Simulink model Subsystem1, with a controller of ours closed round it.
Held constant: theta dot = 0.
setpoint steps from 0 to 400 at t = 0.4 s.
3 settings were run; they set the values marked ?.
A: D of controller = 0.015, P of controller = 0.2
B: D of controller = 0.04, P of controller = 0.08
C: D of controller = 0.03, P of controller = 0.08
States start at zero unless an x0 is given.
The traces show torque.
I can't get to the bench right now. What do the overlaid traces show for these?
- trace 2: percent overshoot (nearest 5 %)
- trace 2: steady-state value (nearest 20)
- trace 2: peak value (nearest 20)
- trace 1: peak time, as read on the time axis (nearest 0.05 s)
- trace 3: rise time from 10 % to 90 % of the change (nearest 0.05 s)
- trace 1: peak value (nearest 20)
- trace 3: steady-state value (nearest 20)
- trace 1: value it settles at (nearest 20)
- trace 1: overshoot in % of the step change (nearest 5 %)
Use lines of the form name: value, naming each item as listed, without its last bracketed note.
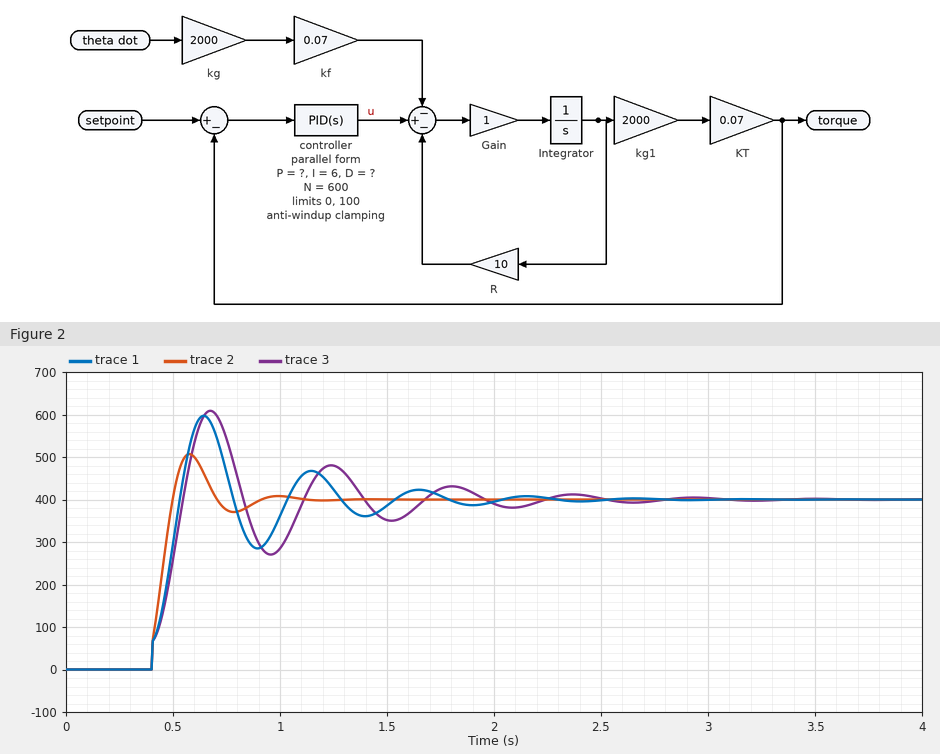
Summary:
trace 2: percent overshoot: 25 %
trace 2: steady-state value: 400
trace 2: peak value: 500
trace 1: peak time, as read on the time axis: 0.65 s
trace 3: rise time from 10 % to 90 % of the change: 0.15 s
trace 1: peak value: 600
trace 3: steady-state value: 400
trace 1: value it settles at: 400
trace 1: overshoot in % of the step change: 50 %
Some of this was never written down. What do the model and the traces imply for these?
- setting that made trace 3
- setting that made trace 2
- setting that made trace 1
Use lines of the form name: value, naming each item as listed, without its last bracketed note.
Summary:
setting that made trace 3: B
setting that made trace 2: A
setting that made trace 1: C
